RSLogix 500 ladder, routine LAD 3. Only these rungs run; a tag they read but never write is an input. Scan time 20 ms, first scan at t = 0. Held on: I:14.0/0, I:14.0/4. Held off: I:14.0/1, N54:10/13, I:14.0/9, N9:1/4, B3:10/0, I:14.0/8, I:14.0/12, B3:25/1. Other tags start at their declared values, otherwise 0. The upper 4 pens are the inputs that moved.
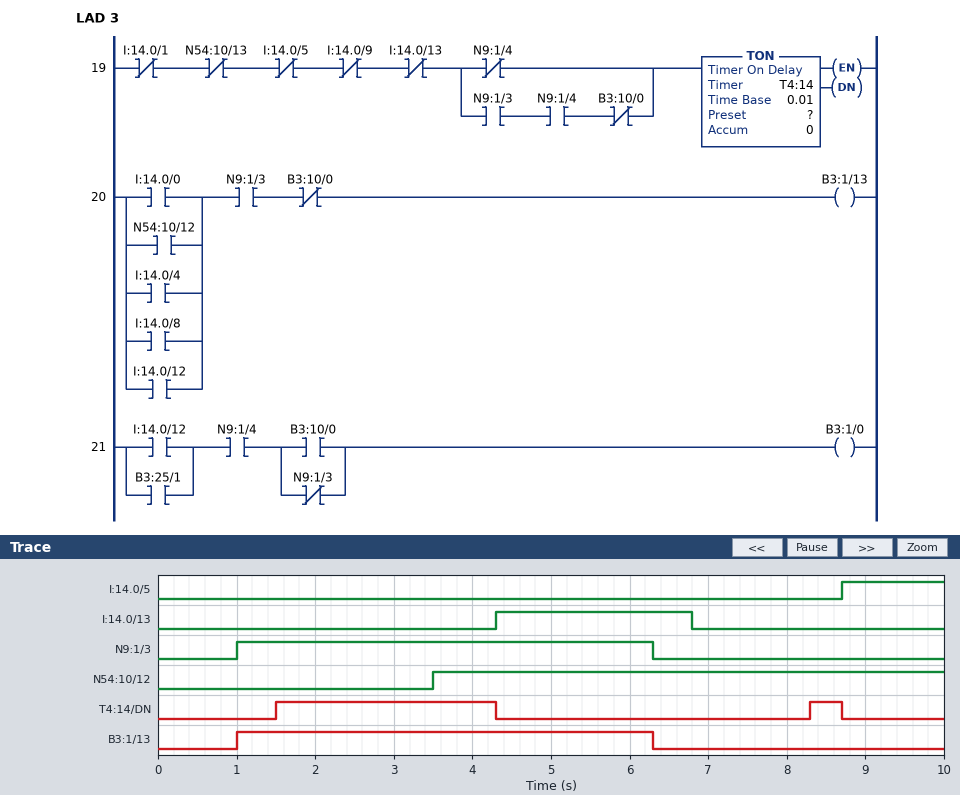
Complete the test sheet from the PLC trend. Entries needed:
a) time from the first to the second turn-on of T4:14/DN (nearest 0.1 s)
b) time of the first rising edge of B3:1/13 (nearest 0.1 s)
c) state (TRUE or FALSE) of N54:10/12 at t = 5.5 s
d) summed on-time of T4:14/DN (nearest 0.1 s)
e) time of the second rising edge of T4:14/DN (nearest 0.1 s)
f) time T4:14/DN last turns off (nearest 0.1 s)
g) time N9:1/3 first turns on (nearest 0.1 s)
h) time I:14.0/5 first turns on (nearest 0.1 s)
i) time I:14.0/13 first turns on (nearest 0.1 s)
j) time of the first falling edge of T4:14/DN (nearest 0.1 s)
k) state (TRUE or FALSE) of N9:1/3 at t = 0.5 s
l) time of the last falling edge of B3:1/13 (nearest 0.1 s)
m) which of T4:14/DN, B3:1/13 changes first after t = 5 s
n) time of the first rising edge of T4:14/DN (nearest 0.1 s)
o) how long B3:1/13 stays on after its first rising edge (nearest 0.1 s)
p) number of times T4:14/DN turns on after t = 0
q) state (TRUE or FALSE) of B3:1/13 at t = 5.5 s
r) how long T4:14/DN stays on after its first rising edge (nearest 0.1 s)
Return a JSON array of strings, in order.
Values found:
["6.8 s", "1.0 s", "TRUE", "3.2 s", "8.3 s", "8.7 s", "1.0 s", "8.7 s", "4.3 s", "4.3 s", "FALSE", "6.3 s", "B3:1/13", "1.5 s", "5.3 s", "2", "TRUE", "2.8 s"]
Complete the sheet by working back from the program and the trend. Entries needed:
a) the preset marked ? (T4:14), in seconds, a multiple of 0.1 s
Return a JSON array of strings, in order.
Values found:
["1.5 s"]
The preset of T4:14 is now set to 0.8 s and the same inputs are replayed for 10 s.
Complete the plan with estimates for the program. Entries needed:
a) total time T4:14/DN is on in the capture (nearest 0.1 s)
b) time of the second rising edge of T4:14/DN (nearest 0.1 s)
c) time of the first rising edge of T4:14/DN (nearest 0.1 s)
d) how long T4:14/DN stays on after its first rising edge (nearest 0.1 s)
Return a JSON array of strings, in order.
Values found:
["4.6 s", "7.6 s", "0.8 s", "3.5 s"]
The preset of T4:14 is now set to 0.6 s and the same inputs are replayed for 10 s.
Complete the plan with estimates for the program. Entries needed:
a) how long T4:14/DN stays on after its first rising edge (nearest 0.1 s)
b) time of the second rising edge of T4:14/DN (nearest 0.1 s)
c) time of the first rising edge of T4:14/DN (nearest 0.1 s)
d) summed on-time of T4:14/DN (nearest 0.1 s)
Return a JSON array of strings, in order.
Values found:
["3.7 s", "7.4 s", "0.6 s", "5.0 s"]
